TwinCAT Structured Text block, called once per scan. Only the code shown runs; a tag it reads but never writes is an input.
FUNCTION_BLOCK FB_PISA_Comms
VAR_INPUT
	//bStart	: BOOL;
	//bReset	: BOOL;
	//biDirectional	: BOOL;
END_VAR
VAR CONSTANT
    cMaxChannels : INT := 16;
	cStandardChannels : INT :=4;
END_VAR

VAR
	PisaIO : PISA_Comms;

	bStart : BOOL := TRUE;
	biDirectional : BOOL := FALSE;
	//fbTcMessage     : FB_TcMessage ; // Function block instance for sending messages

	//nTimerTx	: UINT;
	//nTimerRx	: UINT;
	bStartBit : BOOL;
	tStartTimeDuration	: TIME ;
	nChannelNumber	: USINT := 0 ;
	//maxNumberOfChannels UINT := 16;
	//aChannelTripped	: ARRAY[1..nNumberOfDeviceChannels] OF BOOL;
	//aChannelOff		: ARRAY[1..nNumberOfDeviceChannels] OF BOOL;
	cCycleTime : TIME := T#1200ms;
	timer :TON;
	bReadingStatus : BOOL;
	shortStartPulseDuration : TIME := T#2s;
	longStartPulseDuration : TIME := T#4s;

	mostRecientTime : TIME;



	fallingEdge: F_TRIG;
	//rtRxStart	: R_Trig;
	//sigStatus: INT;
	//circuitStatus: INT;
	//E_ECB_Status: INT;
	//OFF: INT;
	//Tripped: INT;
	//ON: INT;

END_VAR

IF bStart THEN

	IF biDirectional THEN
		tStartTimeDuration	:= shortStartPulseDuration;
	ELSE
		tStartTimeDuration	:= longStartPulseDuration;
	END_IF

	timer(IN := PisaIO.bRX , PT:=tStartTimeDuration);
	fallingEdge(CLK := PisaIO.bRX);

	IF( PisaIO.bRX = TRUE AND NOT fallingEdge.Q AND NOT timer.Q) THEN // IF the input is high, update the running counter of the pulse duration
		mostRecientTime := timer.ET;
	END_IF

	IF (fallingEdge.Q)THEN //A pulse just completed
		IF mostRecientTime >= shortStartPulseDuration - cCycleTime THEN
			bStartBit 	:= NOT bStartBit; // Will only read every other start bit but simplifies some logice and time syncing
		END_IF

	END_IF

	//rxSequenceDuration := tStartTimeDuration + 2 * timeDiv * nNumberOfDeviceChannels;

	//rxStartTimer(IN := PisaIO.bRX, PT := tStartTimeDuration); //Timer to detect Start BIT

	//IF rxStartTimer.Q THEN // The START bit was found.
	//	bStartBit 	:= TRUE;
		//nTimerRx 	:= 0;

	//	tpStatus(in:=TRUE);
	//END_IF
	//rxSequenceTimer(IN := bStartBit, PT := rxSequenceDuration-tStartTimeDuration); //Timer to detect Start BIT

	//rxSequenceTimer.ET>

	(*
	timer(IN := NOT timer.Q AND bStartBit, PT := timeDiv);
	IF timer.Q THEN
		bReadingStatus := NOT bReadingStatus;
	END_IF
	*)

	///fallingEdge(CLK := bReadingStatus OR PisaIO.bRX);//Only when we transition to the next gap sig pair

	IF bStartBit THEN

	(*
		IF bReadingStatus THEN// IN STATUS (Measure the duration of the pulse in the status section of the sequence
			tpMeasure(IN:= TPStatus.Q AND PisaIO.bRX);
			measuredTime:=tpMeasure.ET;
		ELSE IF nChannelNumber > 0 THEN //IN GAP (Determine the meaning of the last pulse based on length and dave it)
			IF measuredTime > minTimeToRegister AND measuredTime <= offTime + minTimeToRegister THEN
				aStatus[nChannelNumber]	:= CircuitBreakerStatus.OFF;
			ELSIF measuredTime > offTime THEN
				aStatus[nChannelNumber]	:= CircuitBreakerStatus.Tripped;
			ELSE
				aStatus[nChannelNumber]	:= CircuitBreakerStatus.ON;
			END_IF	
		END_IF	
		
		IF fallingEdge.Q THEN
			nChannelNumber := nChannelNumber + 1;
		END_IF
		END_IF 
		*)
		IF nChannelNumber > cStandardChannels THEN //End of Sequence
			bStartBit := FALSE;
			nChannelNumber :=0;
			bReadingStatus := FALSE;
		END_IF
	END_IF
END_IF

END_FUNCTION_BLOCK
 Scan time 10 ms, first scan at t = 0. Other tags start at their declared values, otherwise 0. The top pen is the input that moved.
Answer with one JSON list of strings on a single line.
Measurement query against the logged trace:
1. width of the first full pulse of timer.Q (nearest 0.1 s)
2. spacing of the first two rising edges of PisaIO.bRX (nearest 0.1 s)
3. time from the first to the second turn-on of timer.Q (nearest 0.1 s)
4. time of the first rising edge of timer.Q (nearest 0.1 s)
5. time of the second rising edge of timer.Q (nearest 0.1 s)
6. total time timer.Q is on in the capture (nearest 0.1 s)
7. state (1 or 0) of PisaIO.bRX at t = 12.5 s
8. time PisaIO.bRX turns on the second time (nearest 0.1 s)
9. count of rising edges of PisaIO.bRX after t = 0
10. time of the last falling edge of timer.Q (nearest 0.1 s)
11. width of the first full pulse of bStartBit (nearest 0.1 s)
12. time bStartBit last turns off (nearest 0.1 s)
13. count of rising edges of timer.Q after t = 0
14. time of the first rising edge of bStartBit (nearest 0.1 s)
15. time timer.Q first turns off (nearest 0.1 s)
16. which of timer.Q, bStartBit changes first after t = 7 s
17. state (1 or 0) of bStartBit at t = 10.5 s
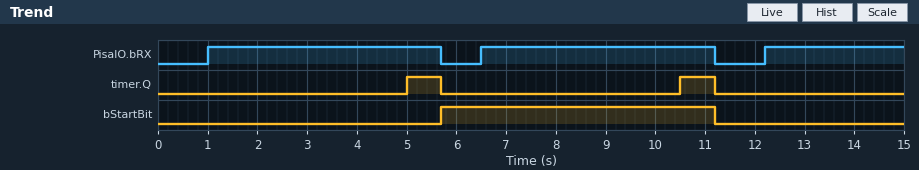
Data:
["0.7 s", "5.5 s", "5.5 s", "5.0 s", "10.5 s", "1.4 s", "1", "6.5 s", "3", "11.2 s", "5.5 s", "11.2 s", "2", "5.7 s", "5.7 s", "timer.Q", "1"]
